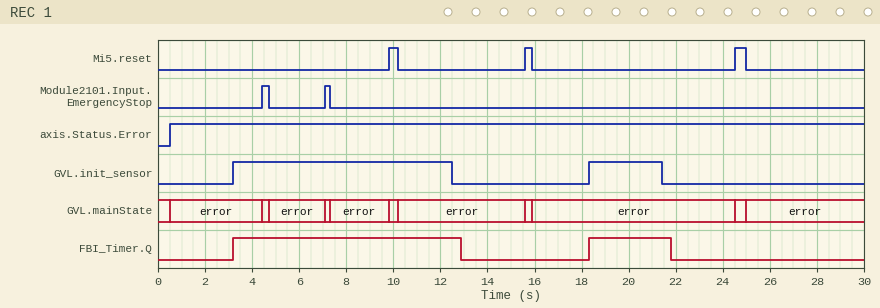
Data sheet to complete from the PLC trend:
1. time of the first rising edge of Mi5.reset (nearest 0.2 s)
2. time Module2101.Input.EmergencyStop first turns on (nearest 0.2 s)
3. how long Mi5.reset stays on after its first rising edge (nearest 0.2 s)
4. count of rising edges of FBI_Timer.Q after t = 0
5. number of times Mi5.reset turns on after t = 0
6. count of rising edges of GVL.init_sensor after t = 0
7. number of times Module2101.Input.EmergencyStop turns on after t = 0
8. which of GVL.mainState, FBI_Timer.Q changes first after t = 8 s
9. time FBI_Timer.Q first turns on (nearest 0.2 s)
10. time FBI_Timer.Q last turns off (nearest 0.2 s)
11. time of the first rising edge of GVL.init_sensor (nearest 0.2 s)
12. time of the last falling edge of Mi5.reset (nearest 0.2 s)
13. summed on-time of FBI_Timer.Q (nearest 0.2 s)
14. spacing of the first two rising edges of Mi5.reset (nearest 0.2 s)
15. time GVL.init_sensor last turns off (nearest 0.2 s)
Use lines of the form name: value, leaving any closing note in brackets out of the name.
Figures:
time of the first rising edge of Mi5.reset: 9.8 s
time Module2101.Input.EmergencyStop first turns on: 4.4 s
how long Mi5.reset stays on after its first rising edge: 0.4 s
count of rising edges of FBI_Timer.Q after t = 0: 2
number of times Mi5.reset turns on after t = 0: 3
count of rising edges of GVL.init_sensor after t = 0: 2
number of times Module2101.Input.EmergencyStop turns on after t = 0: 2
which of GVL.mainState, FBI_Timer.Q changes first after t = 8 s: GVL.mainState
time FBI_Timer.Q first turns on: 3.2 s
time FBI_Timer.Q last turns off: 21.8 s
time of the first rising edge of GVL.init_sensor: 3.2 s
time of the last falling edge of Mi5.reset: 25.0 s
summed on-time of FBI_Timer.Q: 13.2 s
spacing of the first two rising edges of Mi5.reset: 5.8 s
time GVL.init_sensor last turns off: 21.4 s
